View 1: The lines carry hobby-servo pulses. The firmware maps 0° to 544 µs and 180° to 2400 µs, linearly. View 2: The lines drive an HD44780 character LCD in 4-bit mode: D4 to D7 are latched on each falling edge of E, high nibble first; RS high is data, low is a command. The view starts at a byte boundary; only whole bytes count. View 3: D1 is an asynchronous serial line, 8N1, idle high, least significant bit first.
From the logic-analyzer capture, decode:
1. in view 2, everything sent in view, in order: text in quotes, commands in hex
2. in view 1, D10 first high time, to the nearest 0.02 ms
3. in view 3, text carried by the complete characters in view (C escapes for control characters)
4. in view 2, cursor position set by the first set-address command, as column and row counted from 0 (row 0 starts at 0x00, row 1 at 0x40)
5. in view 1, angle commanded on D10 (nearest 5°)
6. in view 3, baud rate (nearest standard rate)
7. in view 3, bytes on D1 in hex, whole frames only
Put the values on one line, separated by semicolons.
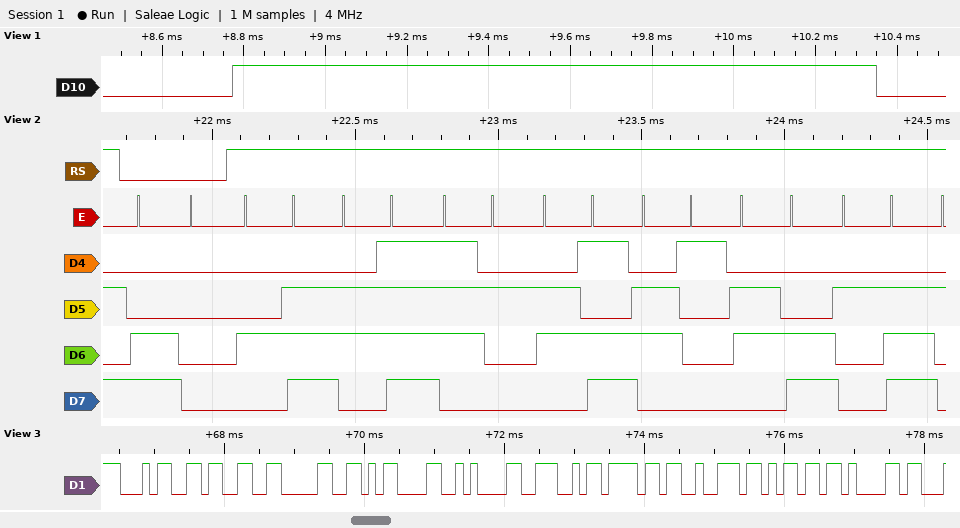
0xC0 "Normal."; 1.58 ms; "430\r\nNorma"; column 0, row 1; 100°; 9600 baud; 34 33 30 0D 0A 4E 6F 72 6D 61
